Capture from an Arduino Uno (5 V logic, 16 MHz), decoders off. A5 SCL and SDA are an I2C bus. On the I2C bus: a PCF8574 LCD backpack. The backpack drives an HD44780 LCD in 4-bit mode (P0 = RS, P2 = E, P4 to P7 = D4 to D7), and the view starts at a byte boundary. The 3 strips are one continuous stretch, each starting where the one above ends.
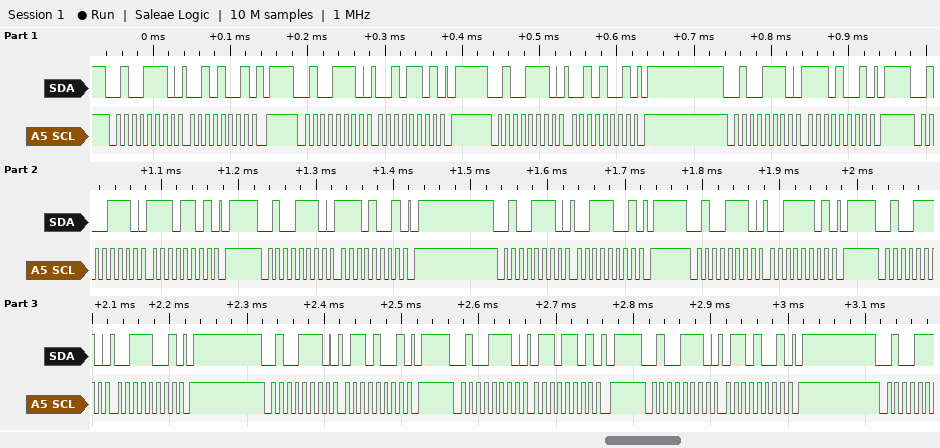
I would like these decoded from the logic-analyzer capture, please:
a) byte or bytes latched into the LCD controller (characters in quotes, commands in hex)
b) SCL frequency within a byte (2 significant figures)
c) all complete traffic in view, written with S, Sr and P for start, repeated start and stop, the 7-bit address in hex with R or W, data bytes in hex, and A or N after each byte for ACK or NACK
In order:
'.' '6'
100 kHz
S 27W A 29 A P S 27W A 2D A P S 27W A 29 A P S 27W A E9 A P S 27W A ED A P S 27W A E9 A P S 27W A 39 A P S 27W A 3D A P S 27W A 39 A P S 27W A 69 A P S 27W A 6D A P S 27W A 69 A P
